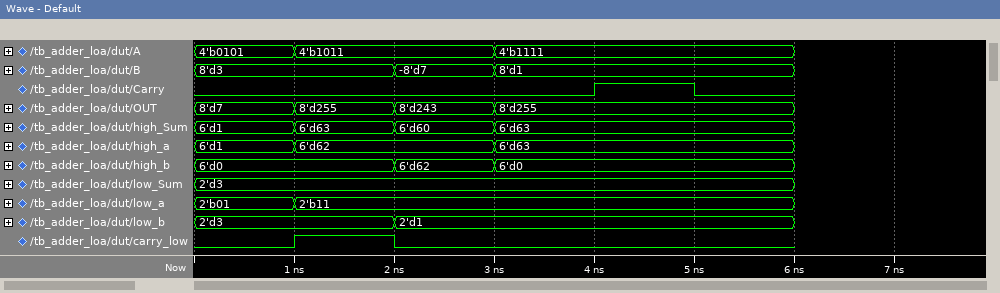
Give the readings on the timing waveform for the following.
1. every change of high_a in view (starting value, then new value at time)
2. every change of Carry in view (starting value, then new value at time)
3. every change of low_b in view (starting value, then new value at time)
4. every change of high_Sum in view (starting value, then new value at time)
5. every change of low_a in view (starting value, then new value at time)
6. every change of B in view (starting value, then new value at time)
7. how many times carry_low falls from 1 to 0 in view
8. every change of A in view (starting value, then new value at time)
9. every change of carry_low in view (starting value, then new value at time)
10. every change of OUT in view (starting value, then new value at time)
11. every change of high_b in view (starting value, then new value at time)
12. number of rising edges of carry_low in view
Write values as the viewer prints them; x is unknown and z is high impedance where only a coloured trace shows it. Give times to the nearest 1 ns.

6'd1, 6'd62 at 1 ns, 6'd63 at 3 ns
0, 1 at 4 ns, 0 at 5 ns
2'd3, 2'd1 at 2 ns
6'd1, 6'd63 at 1 ns, 6'd60 at 2 ns, 6'd63 at 3 ns
2'b01, 2'b11 at 1 ns
8'd3, -8'd7 at 2 ns, 8'd1 at 3 ns
1
4'b0101, 4'b1011 at 1 ns, 4'b1111 at 3 ns
0, 1 at 1 ns, 0 at 2 ns
8'd7, 8'd255 at 1 ns, 8'd243 at 2 ns, 8'd255 at 3 ns
6'd0, 6'd62 at 2 ns, 6'd0 at 3 ns
1
